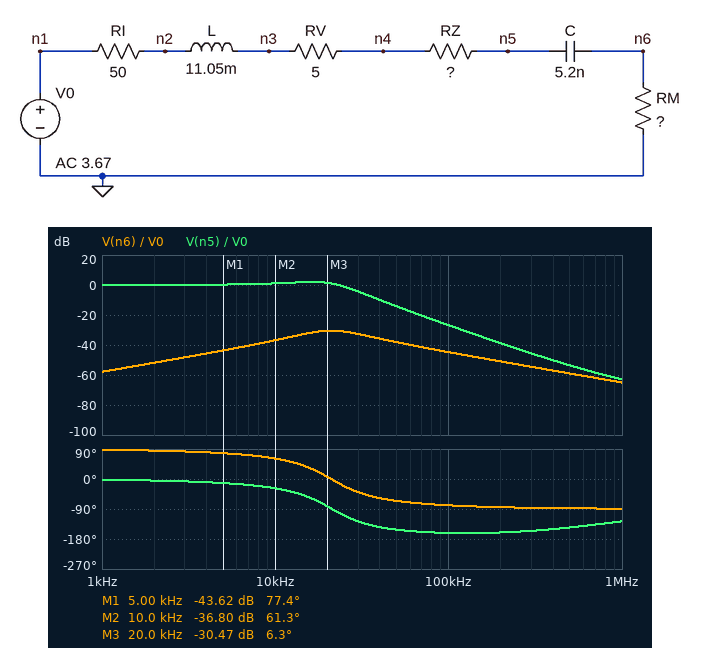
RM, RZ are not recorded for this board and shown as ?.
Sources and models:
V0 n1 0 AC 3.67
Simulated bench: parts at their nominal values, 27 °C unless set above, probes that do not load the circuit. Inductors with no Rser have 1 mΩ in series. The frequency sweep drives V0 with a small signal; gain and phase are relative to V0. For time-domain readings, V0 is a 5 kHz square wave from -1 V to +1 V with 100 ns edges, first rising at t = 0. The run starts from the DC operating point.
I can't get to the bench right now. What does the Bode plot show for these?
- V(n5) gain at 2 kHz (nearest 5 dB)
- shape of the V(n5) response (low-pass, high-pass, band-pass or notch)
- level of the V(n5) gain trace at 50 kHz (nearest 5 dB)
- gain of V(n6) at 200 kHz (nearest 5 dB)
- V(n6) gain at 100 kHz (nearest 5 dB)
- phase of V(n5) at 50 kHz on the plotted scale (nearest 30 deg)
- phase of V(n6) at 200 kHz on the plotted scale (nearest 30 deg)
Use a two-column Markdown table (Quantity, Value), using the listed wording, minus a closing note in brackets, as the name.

| Quantity | Value |
|---|---|
| V(n5) gain at 2 kHz | 0 dB |
| shape of the V(n5) response | low-pass |
| level of the V(n5) gain trace at 50 kHz | -15 dB |
| gain of V(n6) at 200 kHz | -50 dB |
| V(n6) gain at 100 kHz | -45 dB |
| phase of V(n5) at 50 kHz on the plotted scale | -150 deg |
| phase of V(n6) at 200 kHz on the plotted scale | -90 deg |
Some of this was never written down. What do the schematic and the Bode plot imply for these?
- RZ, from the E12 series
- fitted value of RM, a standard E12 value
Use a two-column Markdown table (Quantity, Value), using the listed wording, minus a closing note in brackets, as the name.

| Quantity | Value |
|---|---|
| RZ, from the E12 series | 1.2 kΩ |
| fitted value of RM, a standard E12 value | 39 Ω |
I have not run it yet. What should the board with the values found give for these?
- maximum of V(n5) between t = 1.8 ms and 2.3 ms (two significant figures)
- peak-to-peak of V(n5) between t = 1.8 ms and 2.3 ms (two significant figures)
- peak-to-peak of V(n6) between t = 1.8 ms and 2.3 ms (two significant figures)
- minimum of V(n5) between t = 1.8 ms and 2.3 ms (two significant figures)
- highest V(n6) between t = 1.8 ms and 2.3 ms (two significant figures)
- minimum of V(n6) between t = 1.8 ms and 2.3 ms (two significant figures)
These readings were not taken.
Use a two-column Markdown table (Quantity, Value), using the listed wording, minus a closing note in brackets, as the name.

| Quantity | Value |
|---|---|
| maximum of V(n5) between t = 1.8 ms and 2.3 ms | 1.4 V |
| peak-to-peak of V(n5) between t = 1.8 ms and 2.3 ms | 2.8 V |
| peak-to-peak of V(n6) between t = 1.8 ms and 2.3 ms | 62 mV |
| minimum of V(n5) between t = 1.8 ms and 2.3 ms | -1.4 V |
| highest V(n6) between t = 1.8 ms and 2.3 ms | 31 mV |
| minimum of V(n6) between t = 1.8 ms and 2.3 ms | -31 mV |
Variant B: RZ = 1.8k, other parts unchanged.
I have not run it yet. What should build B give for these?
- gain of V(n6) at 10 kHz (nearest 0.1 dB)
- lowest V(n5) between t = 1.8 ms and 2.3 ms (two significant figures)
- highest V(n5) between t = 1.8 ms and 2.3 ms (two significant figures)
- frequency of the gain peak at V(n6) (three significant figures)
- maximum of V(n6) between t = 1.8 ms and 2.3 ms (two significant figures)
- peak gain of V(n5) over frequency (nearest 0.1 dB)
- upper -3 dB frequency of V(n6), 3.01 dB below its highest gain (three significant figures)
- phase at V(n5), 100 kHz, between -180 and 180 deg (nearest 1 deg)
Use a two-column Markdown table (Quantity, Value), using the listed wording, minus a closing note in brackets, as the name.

| Quantity | Value |
|---|---|
| gain of V(n6) at 10 kHz | -37.8 dB |
| lowest V(n5) between t = 1.8 ms and 2.3 ms | -1.1 V |
| highest V(n5) between t = 1.8 ms and 2.3 ms | 1.1 V |
| frequency of the gain peak at V(n6) | 21.0 kHz |
| maximum of V(n6) between t = 1.8 ms and 2.3 ms | 26 mV |
| peak gain of V(n5) over frequency | 0.1 dB |
| upper -3 dB frequency of V(n6), 3.01 dB below its highest gain | 38.7 kHz |
| phase at V(n5), 100 kHz, between -180 and 180 deg | -157 deg |
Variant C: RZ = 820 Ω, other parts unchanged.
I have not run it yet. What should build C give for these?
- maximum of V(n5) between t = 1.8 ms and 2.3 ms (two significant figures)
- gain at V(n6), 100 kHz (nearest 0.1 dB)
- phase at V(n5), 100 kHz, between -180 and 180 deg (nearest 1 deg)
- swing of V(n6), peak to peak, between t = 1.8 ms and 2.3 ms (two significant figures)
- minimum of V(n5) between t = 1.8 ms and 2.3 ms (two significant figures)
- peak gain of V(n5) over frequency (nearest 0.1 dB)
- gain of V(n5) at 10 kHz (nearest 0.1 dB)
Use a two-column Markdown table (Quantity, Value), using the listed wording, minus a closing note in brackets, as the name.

| Quantity | Value |
|---|---|
| maximum of V(n5) between t = 1.8 ms and 2.3 ms | 1.7 V |
| gain at V(n6), 100 kHz | -44.7 dB |
| phase at V(n5), 100 kHz, between -180 and 180 deg | -165 deg |
| swing of V(n6), peak to peak, between t = 1.8 ms and 2.3 ms | 70 mV |
| minimum of V(n5) between t = 1.8 ms and 2.3 ms | -1.7 V |
| peak gain of V(n5) over frequency | 4.5 dB |
| gain of V(n5) at 10 kHz | 1.6 dB |
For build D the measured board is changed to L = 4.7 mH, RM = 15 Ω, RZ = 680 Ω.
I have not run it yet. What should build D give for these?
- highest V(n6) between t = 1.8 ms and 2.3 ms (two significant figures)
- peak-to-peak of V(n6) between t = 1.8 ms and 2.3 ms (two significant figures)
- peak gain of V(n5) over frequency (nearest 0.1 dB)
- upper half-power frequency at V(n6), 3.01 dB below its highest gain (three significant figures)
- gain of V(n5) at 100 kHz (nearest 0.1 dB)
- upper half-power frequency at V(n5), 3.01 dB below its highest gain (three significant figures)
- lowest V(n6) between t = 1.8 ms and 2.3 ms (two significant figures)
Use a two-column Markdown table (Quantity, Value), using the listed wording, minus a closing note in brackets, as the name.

| Quantity | Value |
|---|---|
| highest V(n6) between t = 1.8 ms and 2.3 ms | 19 mV |
| peak-to-peak of V(n6) between t = 1.8 ms and 2.3 ms | 38 mV |
| peak gain of V(n5) over frequency | 2.8 dB |
| upper half-power frequency at V(n6), 3.01 dB below its highest gain | 47.3 kHz |
| gain of V(n5) at 100 kHz | -19.1 dB |
| upper half-power frequency at V(n5), 3.01 dB below its highest gain | 38.3 kHz |
| lowest V(n6) between t = 1.8 ms and 2.3 ms | -19 mV |
